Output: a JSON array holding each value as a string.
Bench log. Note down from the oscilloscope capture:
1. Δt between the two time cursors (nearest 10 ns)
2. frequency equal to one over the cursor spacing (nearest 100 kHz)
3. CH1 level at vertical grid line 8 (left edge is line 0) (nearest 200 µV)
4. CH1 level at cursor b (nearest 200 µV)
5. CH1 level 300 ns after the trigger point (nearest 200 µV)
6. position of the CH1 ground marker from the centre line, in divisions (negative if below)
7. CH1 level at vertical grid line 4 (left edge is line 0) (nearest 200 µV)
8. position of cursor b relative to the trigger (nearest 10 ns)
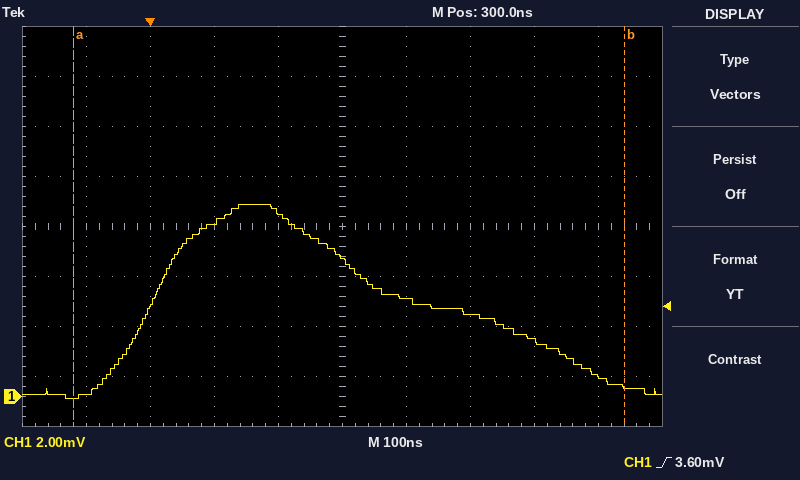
["860 ns", "1.2 MHz", "2.2 mV", "400 µV", "5.6 mV", "-3.4 div", "7.4 mV", "+740 ns"]
